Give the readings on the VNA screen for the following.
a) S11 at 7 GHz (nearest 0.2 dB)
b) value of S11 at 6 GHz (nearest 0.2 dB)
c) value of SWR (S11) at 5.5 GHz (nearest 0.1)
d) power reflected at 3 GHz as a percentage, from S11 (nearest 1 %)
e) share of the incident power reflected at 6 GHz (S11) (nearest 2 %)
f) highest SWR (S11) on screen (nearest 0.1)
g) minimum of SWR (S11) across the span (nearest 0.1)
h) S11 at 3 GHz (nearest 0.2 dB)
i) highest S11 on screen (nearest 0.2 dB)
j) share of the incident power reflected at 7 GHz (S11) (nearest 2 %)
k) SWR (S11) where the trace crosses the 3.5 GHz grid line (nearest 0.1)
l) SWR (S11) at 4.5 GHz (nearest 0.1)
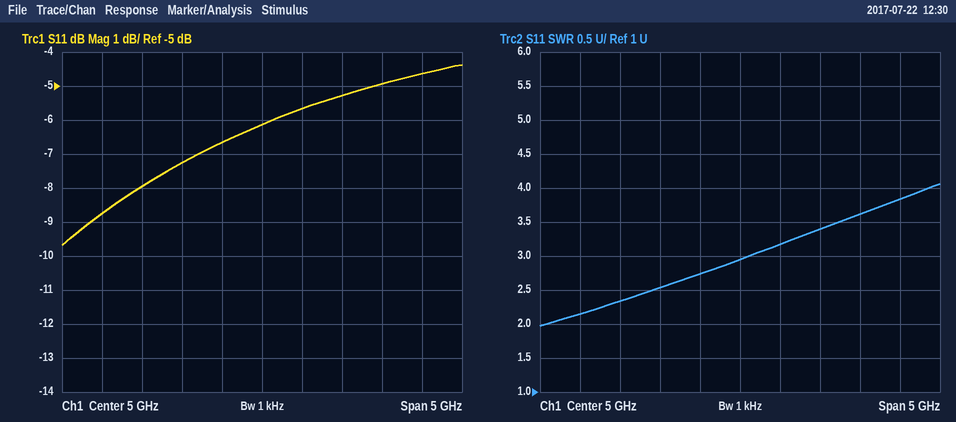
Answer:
-4.6 dB
-5.2 dB
3.2
13 %
30 %
4.1
2.0
-8.8 dB
-4.4 dB
34 %
2.3
2.7
